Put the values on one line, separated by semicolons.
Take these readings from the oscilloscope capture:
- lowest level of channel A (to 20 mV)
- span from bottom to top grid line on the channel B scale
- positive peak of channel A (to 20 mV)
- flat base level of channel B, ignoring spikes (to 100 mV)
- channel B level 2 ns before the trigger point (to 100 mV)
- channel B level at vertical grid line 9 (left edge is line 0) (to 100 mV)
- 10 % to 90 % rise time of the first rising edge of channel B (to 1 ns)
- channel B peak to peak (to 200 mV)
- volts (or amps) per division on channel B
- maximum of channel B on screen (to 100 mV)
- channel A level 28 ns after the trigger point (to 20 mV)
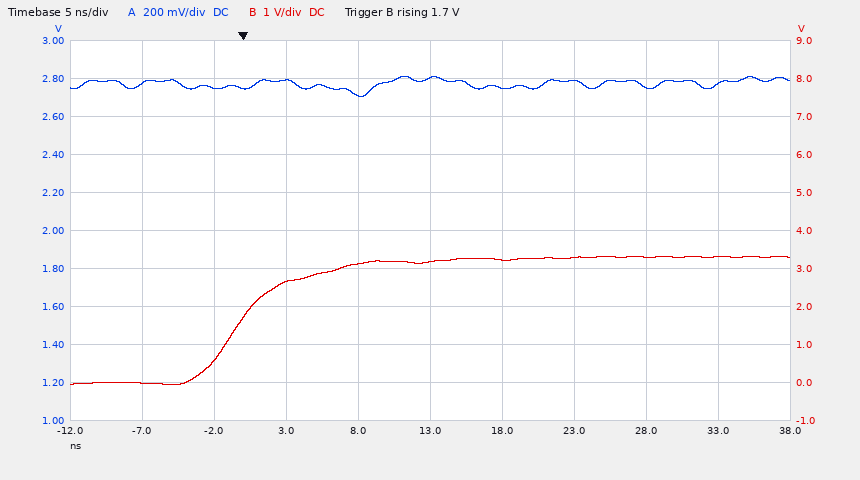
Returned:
2.70 V; 10 V; 2.82 V; 0.0 V; 600 mV; 3.3 V; 9 ns; 3.4 V; 1 V; 3.3 V; 2.76 V
